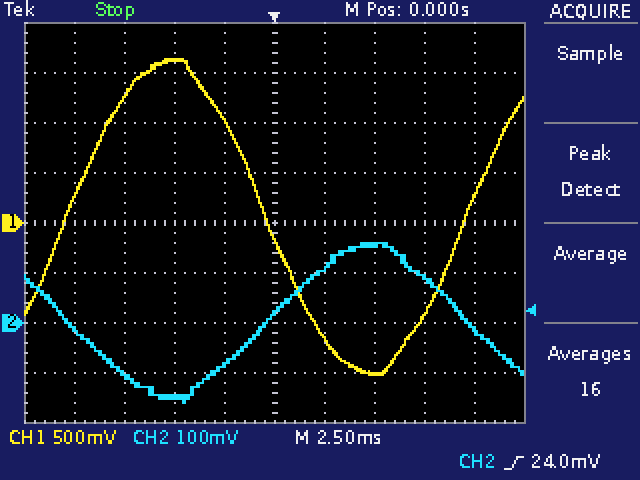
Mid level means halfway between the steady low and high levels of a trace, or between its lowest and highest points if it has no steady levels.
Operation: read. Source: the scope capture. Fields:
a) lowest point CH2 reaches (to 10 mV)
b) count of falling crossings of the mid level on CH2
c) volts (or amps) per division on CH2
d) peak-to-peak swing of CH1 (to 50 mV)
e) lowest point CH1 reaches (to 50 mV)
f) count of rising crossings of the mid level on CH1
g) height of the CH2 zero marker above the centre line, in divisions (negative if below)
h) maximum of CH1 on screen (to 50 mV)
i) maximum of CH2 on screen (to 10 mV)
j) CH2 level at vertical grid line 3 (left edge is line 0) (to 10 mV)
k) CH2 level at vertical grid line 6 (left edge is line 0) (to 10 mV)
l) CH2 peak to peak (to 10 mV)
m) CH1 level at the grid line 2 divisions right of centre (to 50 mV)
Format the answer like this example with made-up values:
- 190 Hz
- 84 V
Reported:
- -160 mV
- 2
- 100 mV
- 3.15 V
- -1.50 V
- 2
- -2.0 div
- 1.65 V
- 160 mV
- -150 mV
- 110 mV
- 320 mV
- -1.50 V
